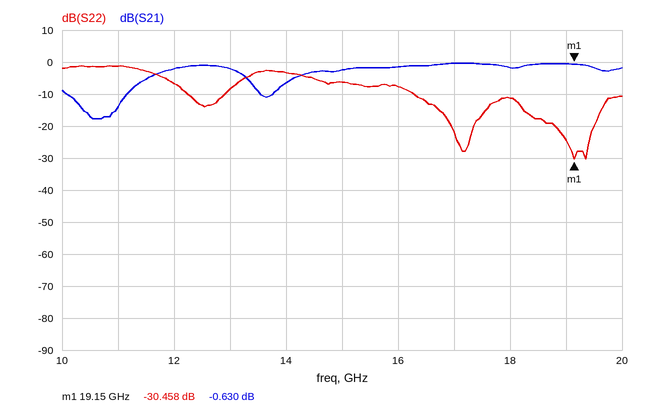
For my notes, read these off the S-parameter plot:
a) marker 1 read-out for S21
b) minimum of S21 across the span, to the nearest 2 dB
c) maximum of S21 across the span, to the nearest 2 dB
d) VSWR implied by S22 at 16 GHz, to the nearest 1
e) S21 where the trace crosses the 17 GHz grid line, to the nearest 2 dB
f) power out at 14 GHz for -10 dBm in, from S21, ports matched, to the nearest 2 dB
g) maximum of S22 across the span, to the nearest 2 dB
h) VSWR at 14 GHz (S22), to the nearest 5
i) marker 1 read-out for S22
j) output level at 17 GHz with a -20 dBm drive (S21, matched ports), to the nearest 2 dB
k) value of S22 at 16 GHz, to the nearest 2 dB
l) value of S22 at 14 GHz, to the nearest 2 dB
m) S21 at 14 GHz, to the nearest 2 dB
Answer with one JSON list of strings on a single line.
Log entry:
["-0.630 dB", "-18 dB", "0 dB", "2", "0 dB", "-16 dBm", "-2 dB", "5", "-30.458 dB", "-20 dBm", "-8 dB", "-4 dB", "-6 dB"]
